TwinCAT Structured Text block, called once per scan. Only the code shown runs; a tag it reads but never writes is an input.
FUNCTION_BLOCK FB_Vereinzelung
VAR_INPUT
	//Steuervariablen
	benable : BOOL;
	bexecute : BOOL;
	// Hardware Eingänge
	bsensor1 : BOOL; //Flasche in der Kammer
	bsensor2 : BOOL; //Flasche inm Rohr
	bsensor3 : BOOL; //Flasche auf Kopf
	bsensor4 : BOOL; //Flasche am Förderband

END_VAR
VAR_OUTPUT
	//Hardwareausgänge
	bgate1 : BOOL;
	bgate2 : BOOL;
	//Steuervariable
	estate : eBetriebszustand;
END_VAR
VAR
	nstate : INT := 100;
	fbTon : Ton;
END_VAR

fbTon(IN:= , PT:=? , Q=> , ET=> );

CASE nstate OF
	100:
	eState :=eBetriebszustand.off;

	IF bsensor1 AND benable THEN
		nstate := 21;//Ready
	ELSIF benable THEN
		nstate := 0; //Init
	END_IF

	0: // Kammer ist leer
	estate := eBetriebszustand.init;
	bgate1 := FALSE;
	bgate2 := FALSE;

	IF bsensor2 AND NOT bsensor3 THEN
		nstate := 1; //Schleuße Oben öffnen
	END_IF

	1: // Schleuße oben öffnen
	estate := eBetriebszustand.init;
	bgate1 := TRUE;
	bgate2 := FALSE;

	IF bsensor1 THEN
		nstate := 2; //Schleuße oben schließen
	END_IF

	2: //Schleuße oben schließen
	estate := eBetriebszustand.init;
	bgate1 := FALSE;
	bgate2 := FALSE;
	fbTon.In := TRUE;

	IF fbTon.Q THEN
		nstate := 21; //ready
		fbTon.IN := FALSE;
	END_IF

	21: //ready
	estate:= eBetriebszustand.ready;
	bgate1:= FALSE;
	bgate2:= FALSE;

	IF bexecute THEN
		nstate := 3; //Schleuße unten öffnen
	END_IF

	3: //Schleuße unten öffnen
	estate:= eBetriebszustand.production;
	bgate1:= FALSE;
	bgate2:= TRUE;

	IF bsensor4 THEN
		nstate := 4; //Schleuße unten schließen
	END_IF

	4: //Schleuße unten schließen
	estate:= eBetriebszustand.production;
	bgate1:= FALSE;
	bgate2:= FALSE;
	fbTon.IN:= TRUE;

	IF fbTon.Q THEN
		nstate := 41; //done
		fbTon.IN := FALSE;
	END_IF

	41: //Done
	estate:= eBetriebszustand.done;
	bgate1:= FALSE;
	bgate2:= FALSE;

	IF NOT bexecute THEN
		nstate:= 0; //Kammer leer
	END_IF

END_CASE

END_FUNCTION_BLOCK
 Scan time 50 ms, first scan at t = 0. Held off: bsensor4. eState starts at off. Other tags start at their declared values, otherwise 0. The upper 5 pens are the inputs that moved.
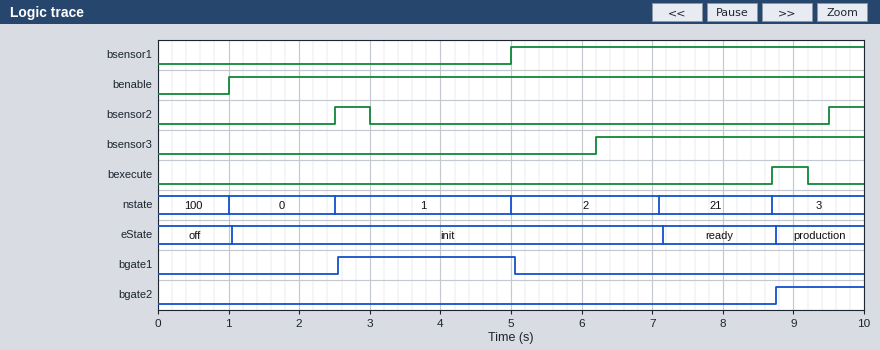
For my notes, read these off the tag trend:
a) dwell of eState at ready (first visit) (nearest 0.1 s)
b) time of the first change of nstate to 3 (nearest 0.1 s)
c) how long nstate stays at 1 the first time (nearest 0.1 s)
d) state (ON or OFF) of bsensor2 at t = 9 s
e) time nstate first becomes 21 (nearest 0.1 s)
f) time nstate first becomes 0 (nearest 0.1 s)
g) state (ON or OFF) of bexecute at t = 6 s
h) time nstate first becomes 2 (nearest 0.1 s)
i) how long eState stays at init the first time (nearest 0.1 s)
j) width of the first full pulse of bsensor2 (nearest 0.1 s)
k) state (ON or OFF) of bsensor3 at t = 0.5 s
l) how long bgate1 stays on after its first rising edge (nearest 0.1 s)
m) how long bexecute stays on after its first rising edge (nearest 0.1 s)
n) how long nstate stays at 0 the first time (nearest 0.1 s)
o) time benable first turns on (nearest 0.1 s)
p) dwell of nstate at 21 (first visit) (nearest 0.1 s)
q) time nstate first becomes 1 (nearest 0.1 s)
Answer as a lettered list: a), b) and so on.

a) 1.6 s
b) 8.7 s
c) 2.5 s
d) OFF
e) 7.1 s
f) 1.0 s
g) OFF
h) 5.0 s
i) 6.1 s
j) 0.5 s
k) OFF
l) 2.5 s
m) 0.5 s
n) 1.5 s
o) 1.0 s
p) 1.6 s
q) 2.5 s
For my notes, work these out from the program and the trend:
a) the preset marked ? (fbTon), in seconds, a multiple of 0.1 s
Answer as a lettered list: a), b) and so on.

a) 2.0 s
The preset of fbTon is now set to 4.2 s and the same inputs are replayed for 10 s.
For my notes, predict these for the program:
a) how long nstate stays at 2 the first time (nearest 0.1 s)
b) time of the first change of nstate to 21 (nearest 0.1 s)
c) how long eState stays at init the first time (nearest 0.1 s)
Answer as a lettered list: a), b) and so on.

a) 4.3 s
b) 9.3 s
c) 8.3 s
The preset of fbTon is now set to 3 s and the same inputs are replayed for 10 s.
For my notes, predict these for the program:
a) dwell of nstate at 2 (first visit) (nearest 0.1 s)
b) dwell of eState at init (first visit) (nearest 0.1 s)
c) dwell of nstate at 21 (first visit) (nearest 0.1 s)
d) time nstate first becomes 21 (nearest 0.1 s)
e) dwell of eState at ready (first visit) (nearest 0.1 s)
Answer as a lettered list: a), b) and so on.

a) 3.1 s
b) 7.1 s
c) 0.6 s
d) 8.1 s
e) 0.6 s
